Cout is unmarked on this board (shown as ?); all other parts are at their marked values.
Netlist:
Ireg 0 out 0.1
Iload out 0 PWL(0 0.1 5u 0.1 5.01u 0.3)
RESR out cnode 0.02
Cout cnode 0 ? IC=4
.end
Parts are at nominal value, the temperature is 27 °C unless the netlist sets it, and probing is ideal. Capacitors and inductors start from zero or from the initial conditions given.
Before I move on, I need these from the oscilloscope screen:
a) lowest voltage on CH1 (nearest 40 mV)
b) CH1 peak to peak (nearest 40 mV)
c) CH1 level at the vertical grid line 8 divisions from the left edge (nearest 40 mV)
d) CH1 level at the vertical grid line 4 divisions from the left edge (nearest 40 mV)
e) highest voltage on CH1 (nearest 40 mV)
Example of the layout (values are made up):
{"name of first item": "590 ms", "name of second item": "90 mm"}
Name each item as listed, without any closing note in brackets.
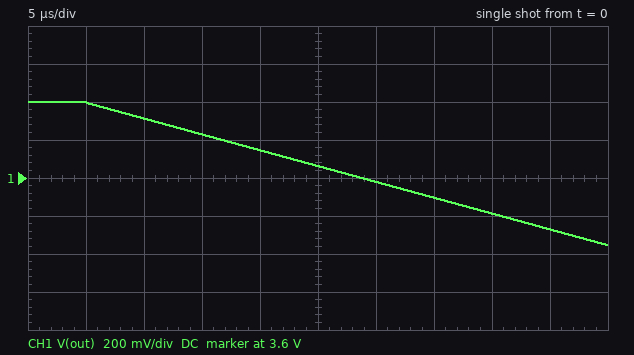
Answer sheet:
{"lowest voltage on CH1": "3.24 V", "CH1 peak to peak": "760 mV", "CH1 level at the vertical grid line 8 divisions from the left edge": "3.40 V", "CH1 level at the vertical grid line 4 divisions from the left edge": "3.76 V", "highest voltage on CH1": "4.00 V"}
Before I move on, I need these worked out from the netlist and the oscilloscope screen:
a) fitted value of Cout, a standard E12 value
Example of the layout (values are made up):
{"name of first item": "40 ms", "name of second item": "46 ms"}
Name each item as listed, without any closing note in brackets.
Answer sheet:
{"fitted value of Cout, a standard E12 value": "12 µF"}
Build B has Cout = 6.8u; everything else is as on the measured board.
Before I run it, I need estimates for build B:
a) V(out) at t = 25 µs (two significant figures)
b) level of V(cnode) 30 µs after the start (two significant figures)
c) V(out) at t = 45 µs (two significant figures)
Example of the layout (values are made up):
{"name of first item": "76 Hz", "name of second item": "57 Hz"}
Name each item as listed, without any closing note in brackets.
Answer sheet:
{"V(out) at t = 25 µs": "3.4 V", "level of V(cnode) 30 µs after the start": "3.3 V", "V(out) at t = 45 µs": "2.8 V"}
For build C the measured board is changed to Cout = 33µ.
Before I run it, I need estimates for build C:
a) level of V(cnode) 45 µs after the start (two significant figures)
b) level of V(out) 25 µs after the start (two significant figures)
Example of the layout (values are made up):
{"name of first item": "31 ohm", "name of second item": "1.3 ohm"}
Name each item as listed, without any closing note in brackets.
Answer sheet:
{"level of V(cnode) 45 µs after the start": "3.8 V", "level of V(out) 25 µs after the start": "3.9 V"}
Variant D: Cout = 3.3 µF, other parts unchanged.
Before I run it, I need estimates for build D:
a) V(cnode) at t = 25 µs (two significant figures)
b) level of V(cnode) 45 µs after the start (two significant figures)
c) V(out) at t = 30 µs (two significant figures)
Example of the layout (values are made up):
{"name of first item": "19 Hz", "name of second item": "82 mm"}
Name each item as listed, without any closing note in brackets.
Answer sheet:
{"V(cnode) at t = 25 µs": "2.8 V", "level of V(cnode) 45 µs after the start": "1.6 V", "V(out) at t = 30 µs": "2.5 V"}
